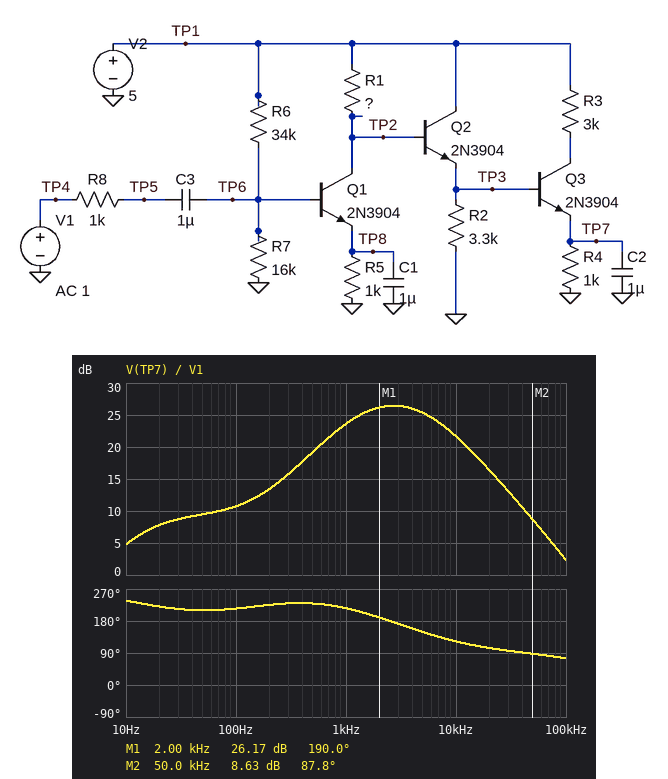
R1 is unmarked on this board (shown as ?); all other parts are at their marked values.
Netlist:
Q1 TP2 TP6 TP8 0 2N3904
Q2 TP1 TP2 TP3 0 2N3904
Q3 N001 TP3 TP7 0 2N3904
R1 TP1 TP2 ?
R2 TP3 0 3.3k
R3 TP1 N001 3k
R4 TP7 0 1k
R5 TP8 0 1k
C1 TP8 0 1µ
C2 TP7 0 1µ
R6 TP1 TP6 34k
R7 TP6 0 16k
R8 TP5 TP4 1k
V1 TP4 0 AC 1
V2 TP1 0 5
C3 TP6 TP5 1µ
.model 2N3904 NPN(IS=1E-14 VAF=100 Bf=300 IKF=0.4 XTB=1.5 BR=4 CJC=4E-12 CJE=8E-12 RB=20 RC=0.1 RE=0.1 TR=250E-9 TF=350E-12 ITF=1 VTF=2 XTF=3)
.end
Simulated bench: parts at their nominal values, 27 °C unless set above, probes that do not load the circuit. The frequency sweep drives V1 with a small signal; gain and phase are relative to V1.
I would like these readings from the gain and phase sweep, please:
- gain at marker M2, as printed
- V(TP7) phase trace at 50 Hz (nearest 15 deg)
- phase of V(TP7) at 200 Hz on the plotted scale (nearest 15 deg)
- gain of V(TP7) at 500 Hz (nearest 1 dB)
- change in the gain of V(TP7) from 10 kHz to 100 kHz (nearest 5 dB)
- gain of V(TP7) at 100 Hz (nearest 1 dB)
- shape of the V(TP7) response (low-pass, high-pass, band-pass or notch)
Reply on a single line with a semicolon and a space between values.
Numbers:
8.63 dB; 210 deg; 225 deg; 19 dB; -20 dB; 11 dB; band-pass
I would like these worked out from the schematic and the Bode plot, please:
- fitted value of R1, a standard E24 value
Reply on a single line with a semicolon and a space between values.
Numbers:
3.9 kΩ
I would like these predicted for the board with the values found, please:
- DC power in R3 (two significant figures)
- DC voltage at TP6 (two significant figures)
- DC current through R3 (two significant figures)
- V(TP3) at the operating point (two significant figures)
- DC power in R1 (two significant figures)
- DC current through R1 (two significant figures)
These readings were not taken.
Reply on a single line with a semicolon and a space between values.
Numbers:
130 µW; 1.6 V; 210 µA; 830 mV; 3.2 mW; 910 µA
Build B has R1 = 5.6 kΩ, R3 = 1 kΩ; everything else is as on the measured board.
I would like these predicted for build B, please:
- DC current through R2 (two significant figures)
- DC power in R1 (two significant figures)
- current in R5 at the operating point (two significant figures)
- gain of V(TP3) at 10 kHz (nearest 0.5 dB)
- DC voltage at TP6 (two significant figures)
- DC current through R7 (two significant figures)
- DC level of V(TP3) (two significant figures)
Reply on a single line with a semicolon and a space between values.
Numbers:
74 µA; 3.1 mW; 760 µA; 1.5 dB; 1.4 V; 88 µA; 240 mV
